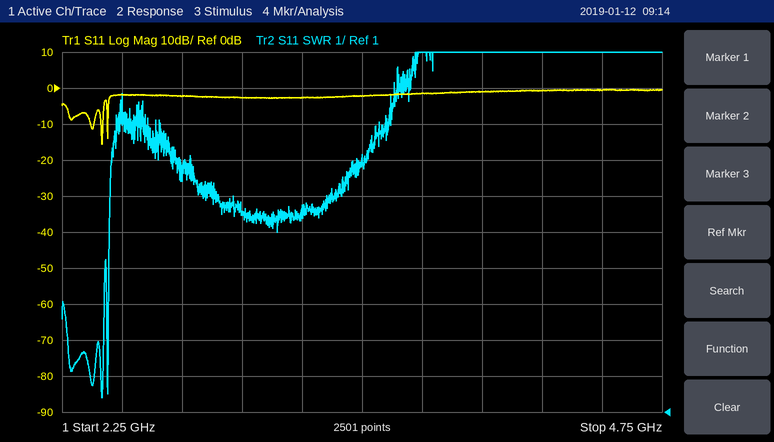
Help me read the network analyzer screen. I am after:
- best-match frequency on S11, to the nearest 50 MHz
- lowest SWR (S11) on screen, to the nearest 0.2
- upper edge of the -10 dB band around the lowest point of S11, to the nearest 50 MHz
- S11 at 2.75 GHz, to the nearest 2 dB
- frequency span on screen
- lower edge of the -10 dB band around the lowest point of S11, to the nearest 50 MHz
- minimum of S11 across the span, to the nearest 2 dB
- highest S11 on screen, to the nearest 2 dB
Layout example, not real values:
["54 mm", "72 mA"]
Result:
["2.40 GHz", "1.4", "2.40 GHz", "-2 dB", "2.5 GHz", "2.40 GHz", "-16 dB", "0 dB"]
